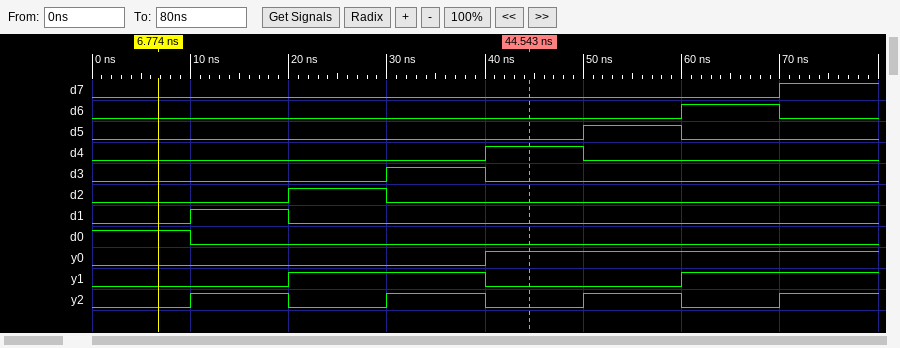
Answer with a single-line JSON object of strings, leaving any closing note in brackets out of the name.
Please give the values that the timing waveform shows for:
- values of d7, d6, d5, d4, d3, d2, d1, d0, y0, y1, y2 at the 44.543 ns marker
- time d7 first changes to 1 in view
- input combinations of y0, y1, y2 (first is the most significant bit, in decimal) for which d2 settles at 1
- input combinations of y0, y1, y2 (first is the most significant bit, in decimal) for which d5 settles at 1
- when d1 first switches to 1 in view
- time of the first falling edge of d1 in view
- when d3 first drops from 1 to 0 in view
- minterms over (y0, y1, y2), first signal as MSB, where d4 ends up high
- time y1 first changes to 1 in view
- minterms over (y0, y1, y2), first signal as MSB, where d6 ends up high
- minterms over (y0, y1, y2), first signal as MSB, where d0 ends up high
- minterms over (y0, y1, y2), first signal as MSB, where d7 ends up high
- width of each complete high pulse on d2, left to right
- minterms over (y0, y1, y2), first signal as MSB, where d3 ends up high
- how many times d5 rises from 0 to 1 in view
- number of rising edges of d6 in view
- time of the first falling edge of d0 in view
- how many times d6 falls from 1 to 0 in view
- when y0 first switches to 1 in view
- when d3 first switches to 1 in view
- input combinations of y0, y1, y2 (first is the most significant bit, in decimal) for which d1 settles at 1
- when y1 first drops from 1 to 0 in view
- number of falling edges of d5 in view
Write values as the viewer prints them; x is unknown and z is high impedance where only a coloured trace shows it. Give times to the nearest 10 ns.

{"values of d7, d6, d5, d4, d3, d2, d1, d0, y0, y1, y2 at the 44.543 ns marker": "d7=0, d6=0, d5=0, d4=1, d3=0, d2=0, d1=0, d0=0, y0=1, y1=0, y2=0", "time d7 first changes to 1 in view": "70 ns", "input combinations of y0, y1, y2 (first is the most significant bit, in decimal) for which d2 settles at 1": "2", "input combinations of y0, y1, y2 (first is the most significant bit, in decimal) for which d5 settles at 1": "5", "when d1 first switches to 1 in view": "10 ns", "time of the first falling edge of d1 in view": "20 ns", "when d3 first drops from 1 to 0 in view": "40 ns", "minterms over (y0, y1, y2), first signal as MSB, where d4 ends up high": "4", "time y1 first changes to 1 in view": "20 ns", "minterms over (y0, y1, y2), first signal as MSB, where d6 ends up high": "6", "minterms over (y0, y1, y2), first signal as MSB, where d0 ends up high": "0", "minterms over (y0, y1, y2), first signal as MSB, where d7 ends up high": "7", "width of each complete high pulse on d2, left to right": "10 ns", "minterms over (y0, y1, y2), first signal as MSB, where d3 ends up high": "3", "how many times d5 rises from 0 to 1 in view": "1", "number of rising edges of d6 in view": "1", "time of the first falling edge of d0 in view": "10 ns", "how many times d6 falls from 1 to 0 in view": "1", "when y0 first switches to 1 in view": "40 ns", "when d3 first switches to 1 in view": "30 ns", "input combinations of y0, y1, y2 (first is the most significant bit, in decimal) for which d1 settles at 1": "1", "when y1 first drops from 1 to 0 in view": "40 ns", "number of falling edges of d5 in view": "1"}
